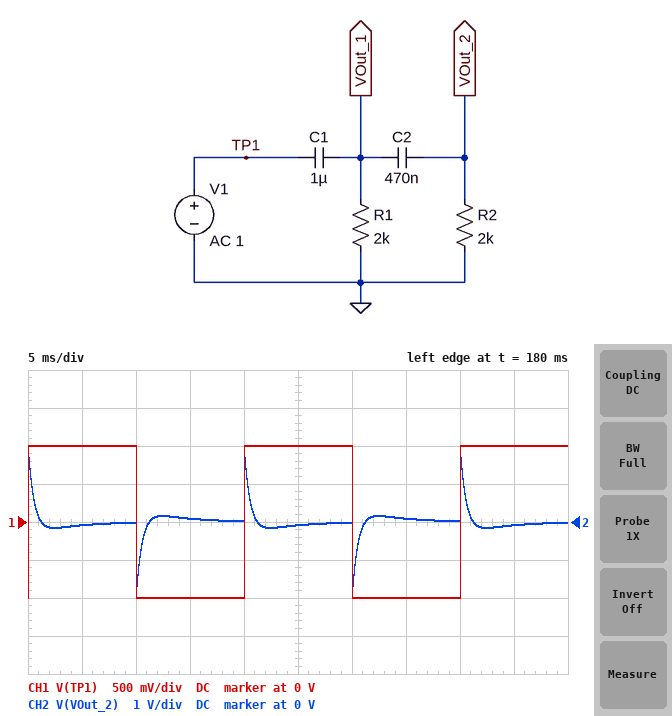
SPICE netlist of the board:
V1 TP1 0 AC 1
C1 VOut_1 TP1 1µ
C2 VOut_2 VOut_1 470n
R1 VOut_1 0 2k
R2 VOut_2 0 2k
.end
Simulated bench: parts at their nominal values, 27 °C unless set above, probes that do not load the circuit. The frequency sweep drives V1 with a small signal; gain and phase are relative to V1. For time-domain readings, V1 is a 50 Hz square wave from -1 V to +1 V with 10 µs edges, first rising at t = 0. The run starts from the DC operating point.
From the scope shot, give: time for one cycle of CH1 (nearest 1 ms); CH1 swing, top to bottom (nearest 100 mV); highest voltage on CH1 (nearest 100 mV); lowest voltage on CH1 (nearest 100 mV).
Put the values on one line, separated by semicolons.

20 ms; 2.0 V; 1.0 V; -1.0 V
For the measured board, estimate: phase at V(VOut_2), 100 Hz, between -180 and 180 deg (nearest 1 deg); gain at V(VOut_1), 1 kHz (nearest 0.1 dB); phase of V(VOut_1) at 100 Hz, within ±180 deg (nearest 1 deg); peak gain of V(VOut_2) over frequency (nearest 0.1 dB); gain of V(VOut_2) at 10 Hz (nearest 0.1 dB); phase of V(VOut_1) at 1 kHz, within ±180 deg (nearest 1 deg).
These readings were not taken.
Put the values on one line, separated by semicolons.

96 deg; -0.2 dB; 37 deg; 0 dB; -42.8 dB; 9 deg
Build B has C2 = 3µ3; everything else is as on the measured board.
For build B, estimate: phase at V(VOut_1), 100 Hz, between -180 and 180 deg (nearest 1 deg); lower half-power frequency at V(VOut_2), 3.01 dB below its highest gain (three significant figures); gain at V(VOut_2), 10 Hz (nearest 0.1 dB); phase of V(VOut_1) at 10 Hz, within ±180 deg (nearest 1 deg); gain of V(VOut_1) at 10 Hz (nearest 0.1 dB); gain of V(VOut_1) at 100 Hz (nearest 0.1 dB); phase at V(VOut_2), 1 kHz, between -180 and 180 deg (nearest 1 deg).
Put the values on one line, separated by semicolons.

53 deg; 173 Hz; -28.2 dB; 67 deg; -19.9 dB; -5.8 dB; 10 deg
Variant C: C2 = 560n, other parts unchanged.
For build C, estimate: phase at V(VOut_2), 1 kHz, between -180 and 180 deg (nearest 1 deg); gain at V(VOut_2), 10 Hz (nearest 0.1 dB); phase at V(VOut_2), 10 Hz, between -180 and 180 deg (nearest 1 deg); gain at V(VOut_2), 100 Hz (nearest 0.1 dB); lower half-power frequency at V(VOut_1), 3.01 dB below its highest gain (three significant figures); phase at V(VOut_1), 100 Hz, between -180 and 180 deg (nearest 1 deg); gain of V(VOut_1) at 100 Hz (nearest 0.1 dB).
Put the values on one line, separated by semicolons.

17 deg; -41.3 dB; 165 deg; -9.6 dB; 178 Hz; 38 deg; -4.8 dB
